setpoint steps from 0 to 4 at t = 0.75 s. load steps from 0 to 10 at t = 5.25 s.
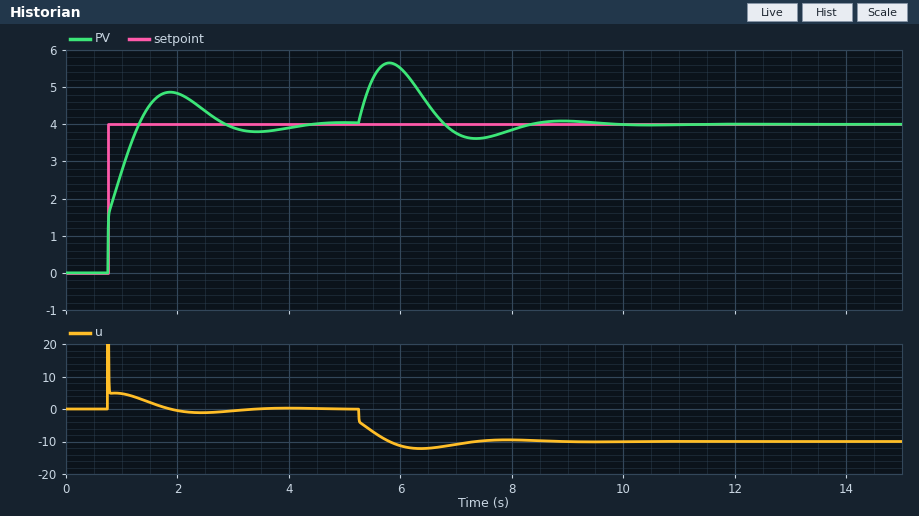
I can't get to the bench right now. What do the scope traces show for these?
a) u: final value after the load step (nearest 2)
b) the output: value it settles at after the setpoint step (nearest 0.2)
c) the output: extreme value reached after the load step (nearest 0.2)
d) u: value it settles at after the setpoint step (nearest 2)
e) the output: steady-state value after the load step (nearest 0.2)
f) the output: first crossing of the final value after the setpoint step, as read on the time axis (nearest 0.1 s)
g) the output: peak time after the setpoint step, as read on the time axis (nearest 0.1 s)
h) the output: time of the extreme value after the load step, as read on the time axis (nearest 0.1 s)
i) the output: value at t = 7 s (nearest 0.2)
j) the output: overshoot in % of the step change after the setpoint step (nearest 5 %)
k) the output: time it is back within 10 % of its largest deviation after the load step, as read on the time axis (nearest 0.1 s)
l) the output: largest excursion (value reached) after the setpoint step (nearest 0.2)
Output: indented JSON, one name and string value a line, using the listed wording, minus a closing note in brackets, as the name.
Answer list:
{
  "u: final value after the load step": "-10",
  "the output: value it settles at after the setpoint step": "4.0",
  "the output: extreme value reached after the load step": "5.6",
  "u: value it settles at after the setpoint step": "0",
  "the output: steady-state value after the load step": "4.0",
  "the output: first crossing of the final value after the setpoint step, as read on the time axis": "1.3 s",
  "the output: peak time after the setpoint step, as read on the time axis": "1.9 s",
  "the output: time of the extreme value after the load step, as read on the time axis": "5.8 s",
  "the output: value at t = 7 s": "3.8",
  "the output: overshoot in % of the step change after the setpoint step": "20 %",
  "the output: time it is back within 10 % of its largest deviation after the load step, as read on the time axis": "8.0 s",
  "the output: largest excursion (value reached) after the setpoint step": "4.8"
}
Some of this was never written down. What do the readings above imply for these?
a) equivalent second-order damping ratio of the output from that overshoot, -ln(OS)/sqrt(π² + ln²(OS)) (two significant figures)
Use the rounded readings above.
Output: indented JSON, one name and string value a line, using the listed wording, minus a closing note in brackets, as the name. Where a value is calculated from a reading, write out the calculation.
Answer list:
{
  "equivalent second-order damping ratio of the output from that overshoot, -ln(OS)/sqrt(π² + ln²(OS))": "ln(0.2) = -1.609; 1.609 / sqrt(9.870 + 2.590) = 0.46"
}
